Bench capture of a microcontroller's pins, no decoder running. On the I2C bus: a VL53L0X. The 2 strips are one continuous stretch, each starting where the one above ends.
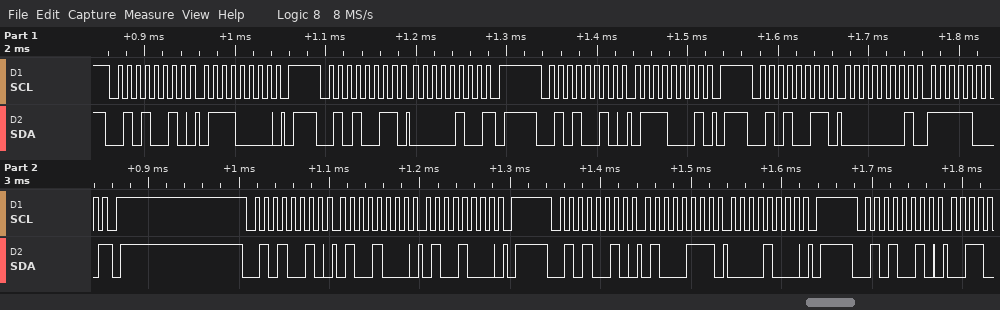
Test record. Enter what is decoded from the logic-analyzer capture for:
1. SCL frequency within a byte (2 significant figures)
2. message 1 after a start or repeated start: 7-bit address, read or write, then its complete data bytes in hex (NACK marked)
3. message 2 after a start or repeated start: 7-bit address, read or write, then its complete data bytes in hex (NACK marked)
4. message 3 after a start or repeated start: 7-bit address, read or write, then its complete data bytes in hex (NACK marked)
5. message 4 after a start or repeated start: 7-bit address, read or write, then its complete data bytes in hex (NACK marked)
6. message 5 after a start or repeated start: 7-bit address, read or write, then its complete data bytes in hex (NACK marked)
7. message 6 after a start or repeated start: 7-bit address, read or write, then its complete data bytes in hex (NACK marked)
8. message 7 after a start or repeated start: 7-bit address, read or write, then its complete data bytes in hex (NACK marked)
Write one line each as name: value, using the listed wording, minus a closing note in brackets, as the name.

SCL frequency within a byte: 100 kHz
message 1 after a start or repeated start: 7-bit address, read or write, then its complete data bytes in hex: 0x29 write: 70
message 2 after a start or repeated start: 7-bit address, read or write, then its complete data bytes in hex: 0x29 read: 04 NACK
message 3 after a start or repeated start: 7-bit address, read or write, then its complete data bytes in hex: 0x29 write: 71
message 4 after a start or repeated start: 7-bit address, read or write, then its complete data bytes in hex: 0x29 read: 01 F8 NACK
message 5 after a start or repeated start: 7-bit address, read or write, then its complete data bytes in hex: 0x29 write: 48 48
message 6 after a start or repeated start: 7-bit address, read or write, then its complete data bytes in hex: 0x29 write: 47 08
message 7 after a start or repeated start: 7-bit address, read or write, then its complete data bytes in hex: 0x29 write
